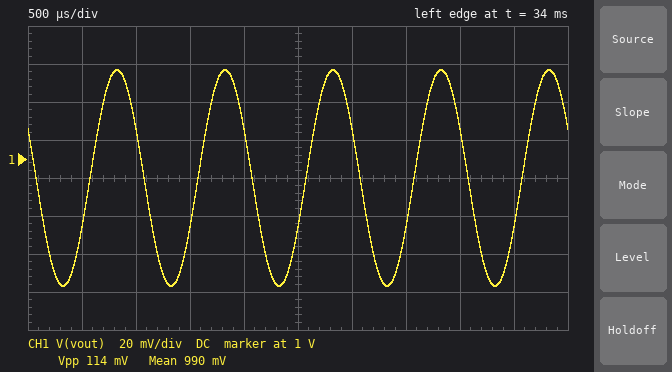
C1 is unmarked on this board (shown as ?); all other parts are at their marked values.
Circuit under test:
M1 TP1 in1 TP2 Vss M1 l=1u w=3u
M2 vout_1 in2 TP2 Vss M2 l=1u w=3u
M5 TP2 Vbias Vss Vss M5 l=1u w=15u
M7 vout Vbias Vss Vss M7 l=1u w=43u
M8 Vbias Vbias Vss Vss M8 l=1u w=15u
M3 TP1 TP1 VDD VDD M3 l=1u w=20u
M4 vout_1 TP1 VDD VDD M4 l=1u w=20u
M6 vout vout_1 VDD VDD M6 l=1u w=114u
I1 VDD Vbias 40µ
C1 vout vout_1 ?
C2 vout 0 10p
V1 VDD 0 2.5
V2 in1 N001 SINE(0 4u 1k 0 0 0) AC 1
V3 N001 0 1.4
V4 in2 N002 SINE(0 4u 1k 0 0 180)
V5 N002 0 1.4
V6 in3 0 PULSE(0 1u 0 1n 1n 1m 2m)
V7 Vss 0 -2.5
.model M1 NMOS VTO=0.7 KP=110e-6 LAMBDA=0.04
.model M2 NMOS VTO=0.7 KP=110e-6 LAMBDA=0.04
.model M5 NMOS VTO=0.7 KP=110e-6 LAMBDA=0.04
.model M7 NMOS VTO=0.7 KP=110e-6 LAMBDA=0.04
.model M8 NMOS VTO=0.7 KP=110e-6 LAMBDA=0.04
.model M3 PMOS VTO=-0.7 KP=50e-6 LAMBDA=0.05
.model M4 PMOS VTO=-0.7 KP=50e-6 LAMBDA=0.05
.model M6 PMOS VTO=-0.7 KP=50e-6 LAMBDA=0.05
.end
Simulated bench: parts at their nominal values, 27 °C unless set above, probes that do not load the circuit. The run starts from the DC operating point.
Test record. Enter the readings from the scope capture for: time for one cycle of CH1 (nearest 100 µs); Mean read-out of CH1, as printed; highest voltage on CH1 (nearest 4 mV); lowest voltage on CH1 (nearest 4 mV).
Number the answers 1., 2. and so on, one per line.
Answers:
1. 1.0 ms
2. 990 mV
3. 1.048 V
4. 932 mV
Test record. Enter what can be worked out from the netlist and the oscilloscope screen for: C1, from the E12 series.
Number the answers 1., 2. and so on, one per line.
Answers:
1. 1.2 pF
